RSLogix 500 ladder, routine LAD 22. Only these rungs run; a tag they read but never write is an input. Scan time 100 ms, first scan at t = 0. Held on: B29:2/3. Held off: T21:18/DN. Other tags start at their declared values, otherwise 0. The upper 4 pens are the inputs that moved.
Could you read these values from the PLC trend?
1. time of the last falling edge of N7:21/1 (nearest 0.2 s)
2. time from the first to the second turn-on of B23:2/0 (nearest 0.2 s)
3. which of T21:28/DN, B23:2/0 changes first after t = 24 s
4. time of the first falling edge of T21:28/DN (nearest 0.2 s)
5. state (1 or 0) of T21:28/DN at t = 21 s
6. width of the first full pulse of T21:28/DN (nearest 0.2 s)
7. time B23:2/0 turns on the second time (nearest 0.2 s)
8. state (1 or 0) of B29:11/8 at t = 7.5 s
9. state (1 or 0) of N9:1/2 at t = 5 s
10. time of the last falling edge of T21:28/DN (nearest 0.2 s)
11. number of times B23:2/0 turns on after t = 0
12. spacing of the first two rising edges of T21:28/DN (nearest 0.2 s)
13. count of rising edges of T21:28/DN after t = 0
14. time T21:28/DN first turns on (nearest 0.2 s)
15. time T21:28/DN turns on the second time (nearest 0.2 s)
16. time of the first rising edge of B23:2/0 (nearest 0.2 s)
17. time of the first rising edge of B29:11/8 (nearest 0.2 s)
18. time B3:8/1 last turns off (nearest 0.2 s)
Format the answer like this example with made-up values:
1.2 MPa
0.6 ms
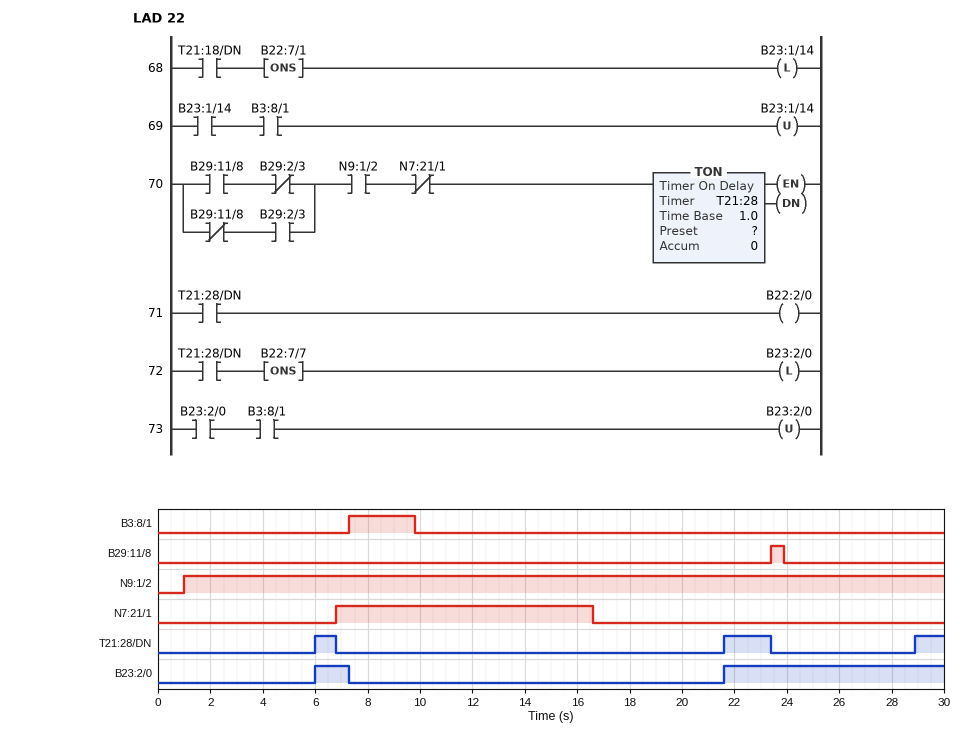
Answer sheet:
16.6 s
15.6 s
T21:28/DN
6.8 s
0
0.8 s
21.6 s
0
1
23.4 s
2
15.6 s
3
6.0 s
21.6 s
6.0 s
23.4 s
9.8 s
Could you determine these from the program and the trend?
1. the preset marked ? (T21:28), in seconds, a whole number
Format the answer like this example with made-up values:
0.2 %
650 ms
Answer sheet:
5 s
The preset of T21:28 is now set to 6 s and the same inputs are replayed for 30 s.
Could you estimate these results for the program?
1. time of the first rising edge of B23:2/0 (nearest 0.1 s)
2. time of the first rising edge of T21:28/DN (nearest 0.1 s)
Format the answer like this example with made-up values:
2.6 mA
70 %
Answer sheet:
22.6 s
22.6 s
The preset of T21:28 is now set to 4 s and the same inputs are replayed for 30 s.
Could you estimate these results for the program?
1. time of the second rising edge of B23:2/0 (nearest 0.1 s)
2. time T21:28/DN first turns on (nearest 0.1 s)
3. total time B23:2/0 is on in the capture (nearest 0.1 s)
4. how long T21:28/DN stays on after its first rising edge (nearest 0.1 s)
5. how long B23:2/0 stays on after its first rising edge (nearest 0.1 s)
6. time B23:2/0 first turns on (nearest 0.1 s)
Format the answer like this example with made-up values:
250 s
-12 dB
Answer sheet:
20.6 s
5.0 s
11.7 s
1.8 s
2.3 s
5.0 s
